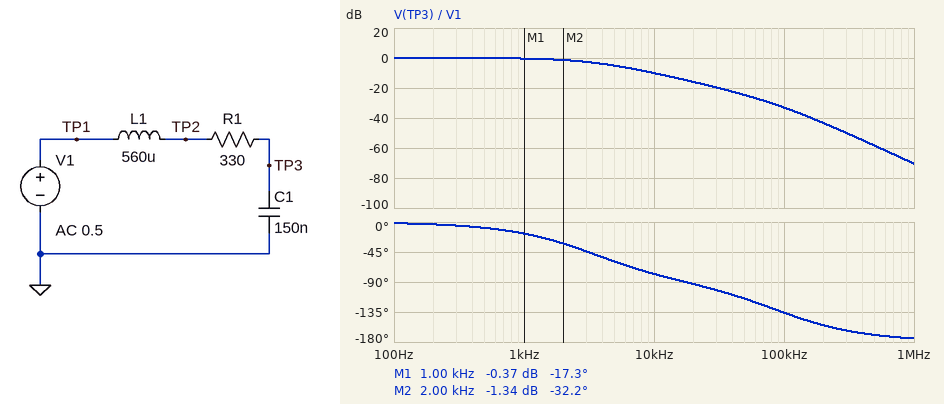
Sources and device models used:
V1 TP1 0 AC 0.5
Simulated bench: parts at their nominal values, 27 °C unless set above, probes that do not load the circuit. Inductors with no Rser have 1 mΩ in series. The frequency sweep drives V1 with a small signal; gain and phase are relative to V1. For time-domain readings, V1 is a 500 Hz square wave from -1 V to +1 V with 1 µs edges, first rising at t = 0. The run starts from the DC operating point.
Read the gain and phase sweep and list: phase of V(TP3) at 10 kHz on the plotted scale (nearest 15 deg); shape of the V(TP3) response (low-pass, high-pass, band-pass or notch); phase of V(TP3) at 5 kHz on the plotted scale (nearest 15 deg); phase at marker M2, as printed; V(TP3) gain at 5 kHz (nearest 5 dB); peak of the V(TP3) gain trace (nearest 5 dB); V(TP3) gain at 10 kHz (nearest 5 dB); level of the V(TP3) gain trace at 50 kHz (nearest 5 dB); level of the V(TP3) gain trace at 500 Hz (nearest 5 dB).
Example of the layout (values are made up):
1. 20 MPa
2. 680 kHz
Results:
1. -75 deg
2. low-pass
3. -60 deg
4. -32.2 deg
5. -5 dB
6. 0 dB
7. -10 dB
8. -25 dB
9. 0 dB
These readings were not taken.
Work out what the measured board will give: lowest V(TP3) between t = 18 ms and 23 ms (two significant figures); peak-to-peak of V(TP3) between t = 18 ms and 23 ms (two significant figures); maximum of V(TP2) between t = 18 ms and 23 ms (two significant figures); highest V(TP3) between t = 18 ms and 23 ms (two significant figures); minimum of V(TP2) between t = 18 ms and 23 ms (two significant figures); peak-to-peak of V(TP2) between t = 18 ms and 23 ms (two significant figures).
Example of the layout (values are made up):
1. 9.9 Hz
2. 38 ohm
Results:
1. -1.0 V
2. 2.0 V
3. 1.1 V
4. 1.0 V
5. -1.1 V
6. 2.1 V
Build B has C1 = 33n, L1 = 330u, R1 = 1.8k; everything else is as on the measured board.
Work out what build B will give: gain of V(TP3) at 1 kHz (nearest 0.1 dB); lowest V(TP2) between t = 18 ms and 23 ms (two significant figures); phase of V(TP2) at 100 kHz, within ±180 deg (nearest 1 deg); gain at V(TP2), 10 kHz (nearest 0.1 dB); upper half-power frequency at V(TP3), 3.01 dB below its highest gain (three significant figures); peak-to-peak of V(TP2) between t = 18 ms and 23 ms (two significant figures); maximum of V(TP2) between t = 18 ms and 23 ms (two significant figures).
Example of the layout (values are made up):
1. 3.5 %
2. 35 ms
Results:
1. -0.6 dB
2. -1.0 V
3. -7 deg
4. 0 dB
5. 2.69 kHz
6. 2.0 V
7. 1.0 V
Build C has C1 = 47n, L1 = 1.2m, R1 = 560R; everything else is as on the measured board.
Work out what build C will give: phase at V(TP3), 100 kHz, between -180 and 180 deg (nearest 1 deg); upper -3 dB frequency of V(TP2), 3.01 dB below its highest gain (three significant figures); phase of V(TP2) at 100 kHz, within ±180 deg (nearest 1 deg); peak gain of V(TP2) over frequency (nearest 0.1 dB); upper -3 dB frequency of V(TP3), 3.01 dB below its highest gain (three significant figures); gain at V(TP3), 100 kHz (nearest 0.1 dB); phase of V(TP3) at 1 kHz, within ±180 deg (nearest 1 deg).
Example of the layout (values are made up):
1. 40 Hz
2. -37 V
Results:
1. -142 deg
2. 72.4 kHz
3. -56 deg
4. 0.5 dB
5. 6.58 kHz
6. -28.6 dB
7. -9 deg
